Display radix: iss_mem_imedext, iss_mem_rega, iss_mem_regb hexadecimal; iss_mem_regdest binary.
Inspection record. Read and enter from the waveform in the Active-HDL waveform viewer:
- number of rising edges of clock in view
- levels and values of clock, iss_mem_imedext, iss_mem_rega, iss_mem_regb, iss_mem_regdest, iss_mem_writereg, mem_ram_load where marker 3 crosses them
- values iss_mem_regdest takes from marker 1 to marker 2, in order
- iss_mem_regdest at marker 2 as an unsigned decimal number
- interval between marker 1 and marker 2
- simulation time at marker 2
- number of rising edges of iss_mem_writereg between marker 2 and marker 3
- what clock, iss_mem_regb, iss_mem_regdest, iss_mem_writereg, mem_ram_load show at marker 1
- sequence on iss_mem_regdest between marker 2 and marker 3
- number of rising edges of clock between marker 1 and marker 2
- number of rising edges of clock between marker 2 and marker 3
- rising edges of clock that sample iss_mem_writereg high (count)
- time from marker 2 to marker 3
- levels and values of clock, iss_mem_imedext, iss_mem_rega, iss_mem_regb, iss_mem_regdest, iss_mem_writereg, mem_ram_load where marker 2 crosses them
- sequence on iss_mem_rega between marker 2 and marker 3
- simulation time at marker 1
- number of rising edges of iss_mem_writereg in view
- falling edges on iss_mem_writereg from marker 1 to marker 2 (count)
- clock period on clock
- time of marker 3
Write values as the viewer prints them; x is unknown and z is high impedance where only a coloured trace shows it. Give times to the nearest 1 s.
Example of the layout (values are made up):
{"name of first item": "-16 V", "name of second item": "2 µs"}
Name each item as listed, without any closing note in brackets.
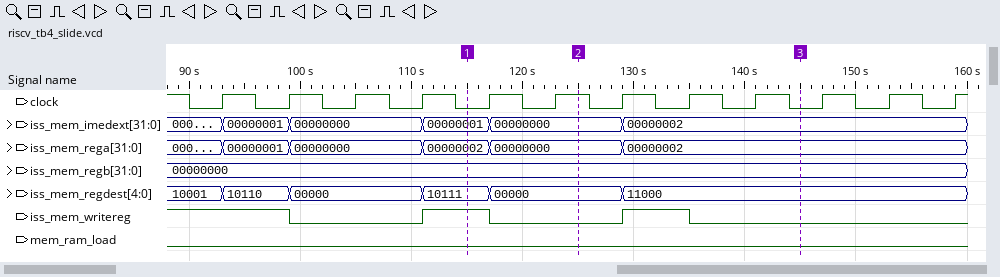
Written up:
{"number of rising edges of clock in view": "12", "levels and values of clock, iss_mem_imedext, iss_mem_rega, iss_mem_regb, iss_mem_regdest, iss_mem_writereg, mem_ram_load where marker 3 crosses them": "clock=0, iss_mem_imedext=00000002, iss_mem_rega=00000002, iss_mem_regb=00000000, iss_mem_regdest=11000, iss_mem_writereg=0, mem_ram_load=0", "values iss_mem_regdest takes from marker 1 to marker 2, in order": "10111, 00000", "iss_mem_regdest at marker 2 as an unsigned decimal number": "0", "interval between marker 1 and marker 2": "10 s", "simulation time at marker 2": "125 s", "number of rising edges of iss_mem_writereg between marker 2 and marker 3": "1", "what clock, iss_mem_regb, iss_mem_regdest, iss_mem_writereg, mem_ram_load show at marker 1": "clock=0, iss_mem_regb=00000000, iss_mem_regdest=10111, iss_mem_writereg=1, mem_ram_load=0", "sequence on iss_mem_regdest between marker 2 and marker 3": "00000, 11000", "number of rising edges of clock between marker 1 and marker 2": "2", "number of rising edges of clock between marker 2 and marker 3": "3", "rising edges of clock that sample iss_mem_writereg high": "4", "time from marker 2 to marker 3": "20 s", "levels and values of clock, iss_mem_imedext, iss_mem_rega, iss_mem_regb, iss_mem_regdest, iss_mem_writereg, mem_ram_load where marker 2 crosses them": "clock=1, iss_mem_imedext=00000000, iss_mem_rega=00000000, iss_mem_regb=00000000, iss_mem_regdest=00000, iss_mem_writereg=0, mem_ram_load=0", "sequence on iss_mem_rega between marker 2 and marker 3": "00000000, 00000002", "simulation time at marker 1": "115 s", "number of rising edges of iss_mem_writereg in view": "2", "falling edges on iss_mem_writereg from marker 1 to marker 2": "1", "clock period on clock": "6 s", "time of marker 3": "145 s"}
